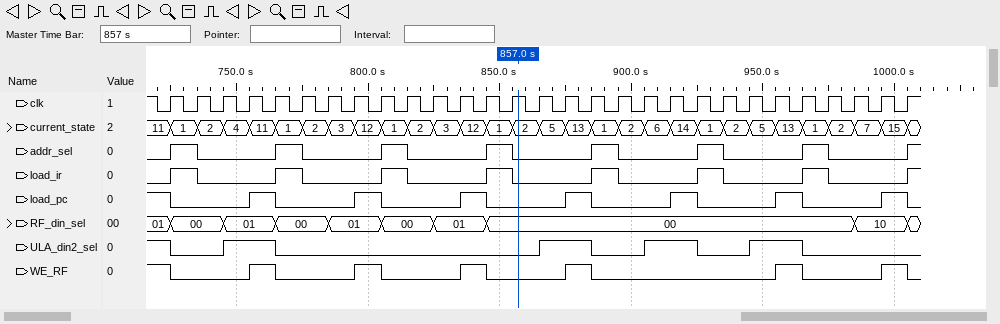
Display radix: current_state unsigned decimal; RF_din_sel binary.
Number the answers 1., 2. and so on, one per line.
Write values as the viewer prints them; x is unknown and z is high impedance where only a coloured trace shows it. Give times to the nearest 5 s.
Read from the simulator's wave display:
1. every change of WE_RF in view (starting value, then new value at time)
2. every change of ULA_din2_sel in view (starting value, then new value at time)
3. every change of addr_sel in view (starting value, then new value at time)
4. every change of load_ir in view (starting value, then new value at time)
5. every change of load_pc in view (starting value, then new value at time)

1. 1, 0 at 725 s, 1 at 755 s, 0 at 765 s, 1 at 795 s, 0 at 805 s, 1 at 835 s, 0 at 845 s, 1 at 875 s, 0 at 885 s, 1 at 955 s, 0 at 965 s, 1 at 995 s, 0 at 1005 s
2. 1, 0 at 725 s, 1 at 745 s, 0 at 765 s, 1 at 865 s, 0 at 885 s, 1 at 905 s, 0 at 925 s, 1 at 945 s, 0 at 965 s
3. 0, 1 at 725 s, 0 at 735 s, 1 at 765 s, 0 at 775 s, 1 at 805 s, 0 at 815 s, 1 at 845 s, 0 at 855 s, 1 at 885 s, 0 at 895 s, 1 at 925 s, 0 at 935 s, 1 at 965 s, 0 at 975 s, 1 at 1005 s
4. 0, 1 at 725 s, 0 at 735 s, 1 at 765 s, 0 at 775 s, 1 at 805 s, 0 at 815 s, 1 at 845 s, 0 at 855 s, 1 at 885 s, 0 at 895 s, 1 at 925 s, 0 at 935 s, 1 at 965 s, 0 at 975 s, 1 at 1005 s
5. 1, 0 at 725 s, 1 at 755 s, 0 at 765 s, 1 at 795 s, 0 at 805 s, 1 at 835 s, 0 at 845 s, 1 at 875 s, 0 at 885 s, 1 at 915 s, 0 at 925 s, 1 at 955 s, 0 at 965 s, 1 at 995 s, 0 at 1005 s
